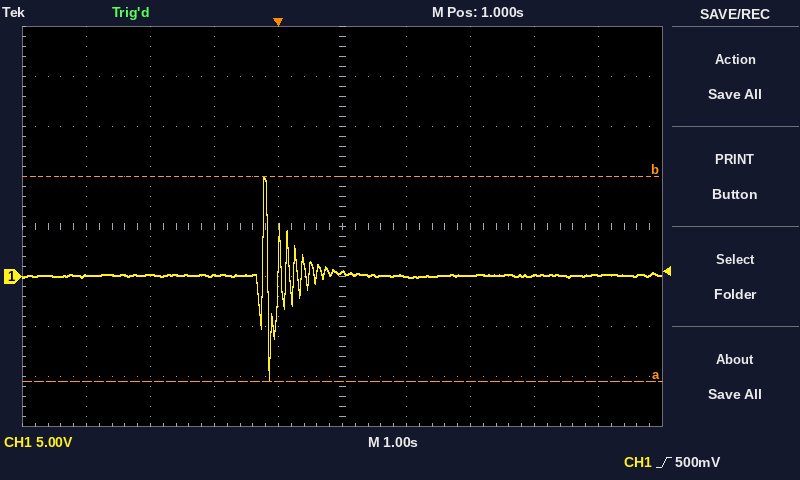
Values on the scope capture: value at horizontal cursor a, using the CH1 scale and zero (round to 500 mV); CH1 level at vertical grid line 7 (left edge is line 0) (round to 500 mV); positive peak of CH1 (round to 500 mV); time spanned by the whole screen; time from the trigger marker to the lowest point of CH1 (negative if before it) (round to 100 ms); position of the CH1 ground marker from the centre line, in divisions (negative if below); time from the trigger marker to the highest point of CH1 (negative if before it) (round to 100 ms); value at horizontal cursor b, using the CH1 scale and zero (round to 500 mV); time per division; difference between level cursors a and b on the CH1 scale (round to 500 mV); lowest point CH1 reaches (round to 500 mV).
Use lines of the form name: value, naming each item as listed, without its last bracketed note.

value at horizontal cursor a, using the CH1 scale and zero: -10.5 V
CH1 level at vertical grid line 7 (left edge is line 0): 0.0 V
positive peak of CH1: 10.0 V
time spanned by the whole screen: 10 s
time from the trigger marker to the lowest point of CH1 (negative if before it): -100 ms
position of the CH1 ground marker from the centre line, in divisions: -1.0 div
time from the trigger marker to the highest point of CH1 (negative if before it): -200 ms
value at horizontal cursor b, using the CH1 scale and zero: 10.0 V
time per division: 1 s
difference between level cursors a and b on the CH1 scale: 20.5 V
lowest point CH1 reaches: -10.5 V
